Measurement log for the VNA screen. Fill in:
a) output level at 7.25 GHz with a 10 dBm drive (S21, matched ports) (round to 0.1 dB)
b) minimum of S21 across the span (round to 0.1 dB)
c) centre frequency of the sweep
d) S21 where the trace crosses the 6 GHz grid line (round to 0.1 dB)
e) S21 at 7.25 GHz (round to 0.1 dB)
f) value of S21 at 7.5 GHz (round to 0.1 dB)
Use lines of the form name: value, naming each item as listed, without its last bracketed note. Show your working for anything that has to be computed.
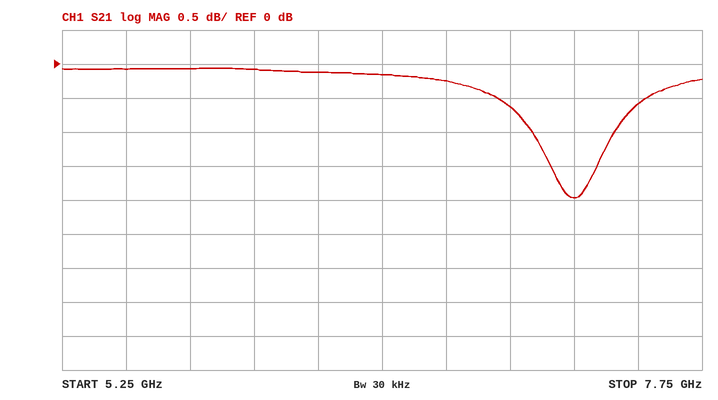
output level at 7.25 GHz with a 10 dBm drive (S21, matched ports): 10 dBm + (-2.0 dB) = 8.0 dBm
minimum of S21 across the span: -2.0 dB
centre frequency of the sweep: 6.5 GHz
S21 where the trace crosses the 6 GHz grid line: -0.1 dB
S21 at 7.25 GHz: -2.0 dB
value of S21 at 7.5 GHz: -0.6 dB
